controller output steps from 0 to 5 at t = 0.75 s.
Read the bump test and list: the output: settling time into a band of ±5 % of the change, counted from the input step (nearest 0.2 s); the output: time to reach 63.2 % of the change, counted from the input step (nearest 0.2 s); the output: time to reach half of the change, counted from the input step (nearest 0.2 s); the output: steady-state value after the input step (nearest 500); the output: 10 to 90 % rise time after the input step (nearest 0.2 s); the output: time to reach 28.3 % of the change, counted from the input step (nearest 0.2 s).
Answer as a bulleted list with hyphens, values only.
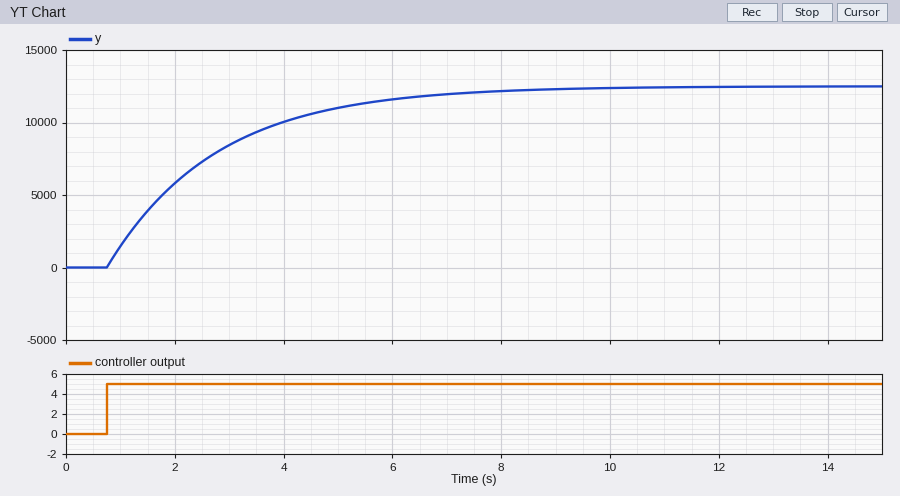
- 6.0 s
- 2.0 s
- 1.4 s
- 12500
- 4.4 s
- 0.6 s
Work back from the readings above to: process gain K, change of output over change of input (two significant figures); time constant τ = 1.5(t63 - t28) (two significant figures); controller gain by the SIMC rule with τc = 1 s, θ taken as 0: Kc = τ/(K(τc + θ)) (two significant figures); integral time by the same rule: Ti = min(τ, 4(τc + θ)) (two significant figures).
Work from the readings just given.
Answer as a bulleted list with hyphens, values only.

- 2500
- 2.1 s
- 0.00084
- 2.1 s
